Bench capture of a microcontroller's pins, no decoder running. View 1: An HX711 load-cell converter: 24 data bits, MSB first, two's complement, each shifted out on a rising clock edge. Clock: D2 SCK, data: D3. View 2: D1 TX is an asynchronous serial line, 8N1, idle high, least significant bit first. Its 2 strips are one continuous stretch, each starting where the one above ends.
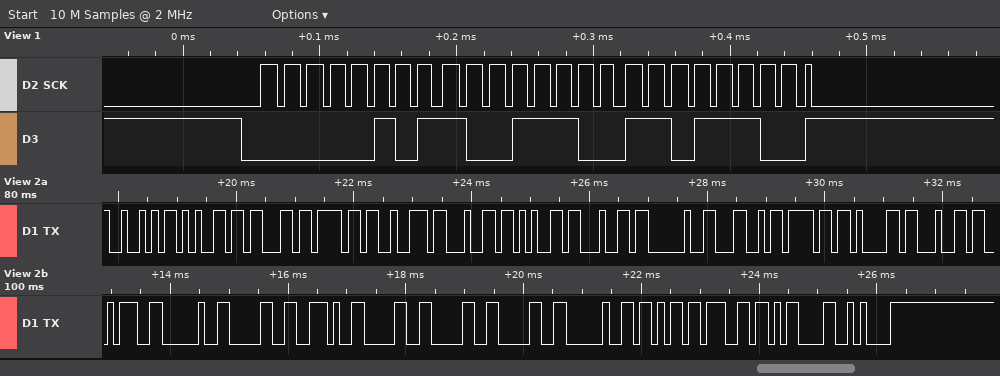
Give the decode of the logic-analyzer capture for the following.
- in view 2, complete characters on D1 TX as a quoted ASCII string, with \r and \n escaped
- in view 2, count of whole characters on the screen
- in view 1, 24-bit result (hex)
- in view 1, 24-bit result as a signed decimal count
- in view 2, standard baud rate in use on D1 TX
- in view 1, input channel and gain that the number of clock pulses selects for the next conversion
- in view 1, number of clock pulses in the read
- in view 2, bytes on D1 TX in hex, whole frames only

"Recorded Load: 0.000 kg\r\n"
25
0x059CDC
367836
9600 baud
channel A, gain 128
25
52 65 63 6F 72 64 65 64 20 4C 6F 61 64 3A 20 30 2E 30 30 30 20 6B 67 0D 0A
